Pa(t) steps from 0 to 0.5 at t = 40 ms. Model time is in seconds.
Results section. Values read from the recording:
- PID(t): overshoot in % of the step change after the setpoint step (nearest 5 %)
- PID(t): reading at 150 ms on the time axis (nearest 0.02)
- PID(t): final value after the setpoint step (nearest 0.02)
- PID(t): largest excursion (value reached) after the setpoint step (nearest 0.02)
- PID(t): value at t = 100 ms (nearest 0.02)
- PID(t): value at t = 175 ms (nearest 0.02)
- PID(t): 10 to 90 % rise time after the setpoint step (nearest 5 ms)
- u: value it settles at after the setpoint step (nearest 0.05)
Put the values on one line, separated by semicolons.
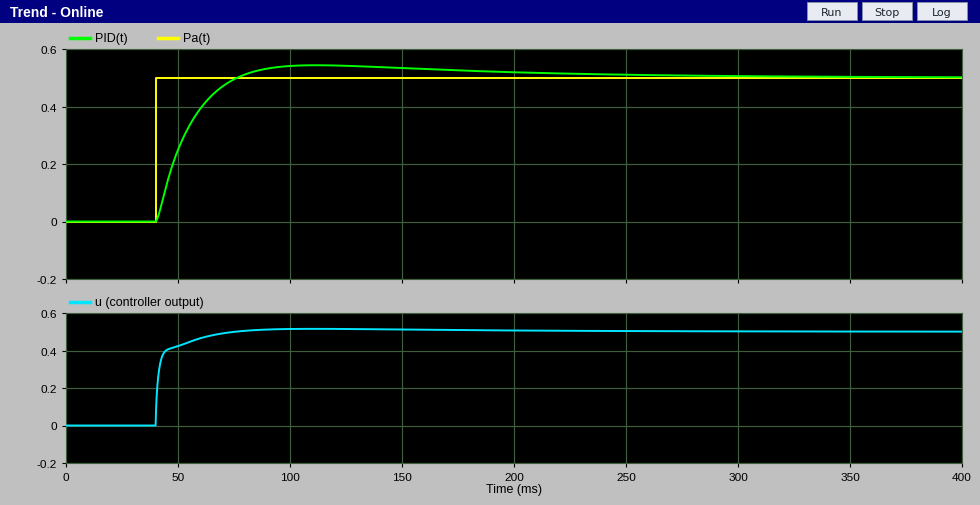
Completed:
10 %; 0.54; 0.50; 0.54; 0.54; 0.52; 25 ms; 0.50
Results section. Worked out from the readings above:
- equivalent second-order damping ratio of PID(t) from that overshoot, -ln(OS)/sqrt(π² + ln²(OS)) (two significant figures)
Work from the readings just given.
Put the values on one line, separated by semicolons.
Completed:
0.59
